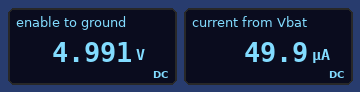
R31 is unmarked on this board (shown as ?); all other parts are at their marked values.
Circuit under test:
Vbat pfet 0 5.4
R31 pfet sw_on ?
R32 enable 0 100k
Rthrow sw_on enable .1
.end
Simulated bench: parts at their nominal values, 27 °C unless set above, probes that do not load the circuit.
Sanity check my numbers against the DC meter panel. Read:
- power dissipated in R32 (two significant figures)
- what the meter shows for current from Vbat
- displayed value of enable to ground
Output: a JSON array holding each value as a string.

["250 µW", "49.9 µA", "4.991 V"]
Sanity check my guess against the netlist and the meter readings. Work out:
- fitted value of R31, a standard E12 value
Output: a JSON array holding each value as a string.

["8.2 kΩ"]
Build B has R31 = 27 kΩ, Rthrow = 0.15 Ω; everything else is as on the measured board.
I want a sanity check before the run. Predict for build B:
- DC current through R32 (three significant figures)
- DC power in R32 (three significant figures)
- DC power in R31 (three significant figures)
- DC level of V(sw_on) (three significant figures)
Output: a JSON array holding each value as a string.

["42.5 µA", "181 µW", "48.8 µW", "4.25 V"]
